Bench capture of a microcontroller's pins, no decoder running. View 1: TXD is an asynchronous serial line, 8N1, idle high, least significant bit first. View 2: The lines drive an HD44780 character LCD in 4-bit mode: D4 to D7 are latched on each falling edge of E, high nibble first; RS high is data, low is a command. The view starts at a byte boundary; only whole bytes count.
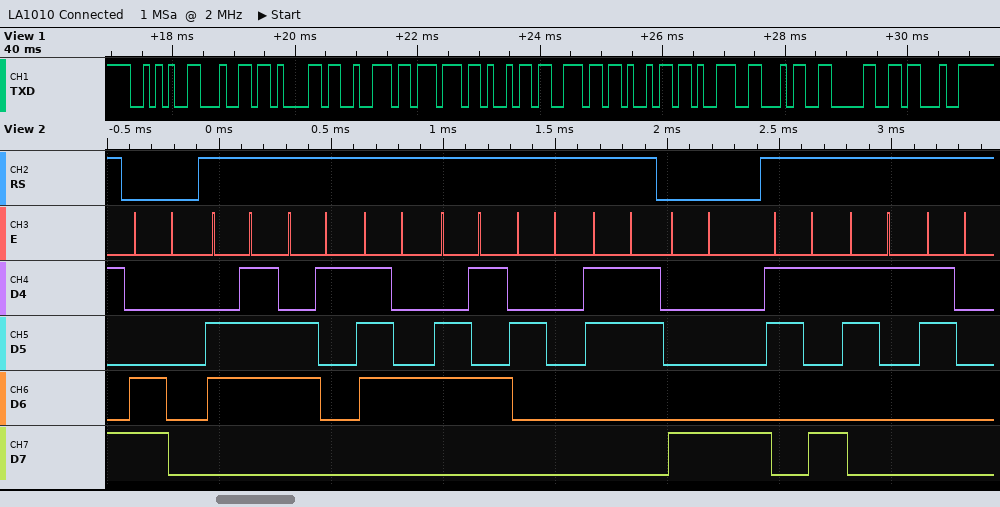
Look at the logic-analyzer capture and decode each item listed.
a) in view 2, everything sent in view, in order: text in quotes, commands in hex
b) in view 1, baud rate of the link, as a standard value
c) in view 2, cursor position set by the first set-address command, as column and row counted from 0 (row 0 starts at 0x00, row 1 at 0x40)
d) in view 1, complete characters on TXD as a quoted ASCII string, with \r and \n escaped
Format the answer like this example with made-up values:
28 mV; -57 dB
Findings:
0xC0 "gate 3" 0x88 "910"; 9600 baud; column 0, row 1; "*darwini940#"
